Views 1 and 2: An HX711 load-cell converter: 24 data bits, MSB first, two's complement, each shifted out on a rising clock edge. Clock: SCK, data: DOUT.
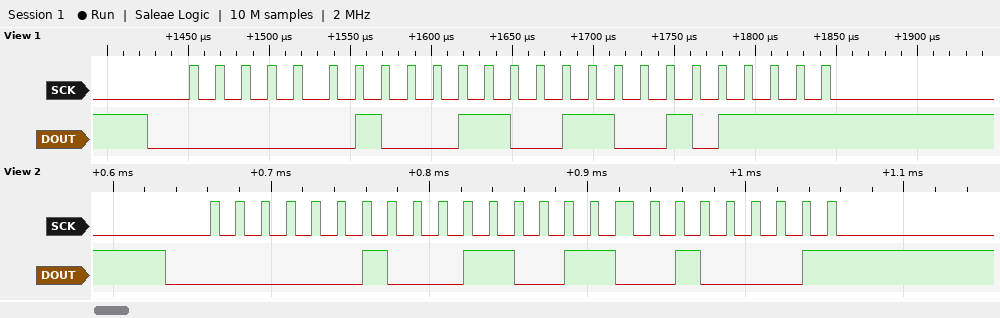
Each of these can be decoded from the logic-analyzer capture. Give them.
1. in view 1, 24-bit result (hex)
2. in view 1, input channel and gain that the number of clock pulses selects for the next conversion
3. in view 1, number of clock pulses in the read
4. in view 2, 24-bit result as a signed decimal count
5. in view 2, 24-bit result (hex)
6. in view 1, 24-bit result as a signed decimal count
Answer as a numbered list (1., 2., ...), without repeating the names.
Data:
1. 0x02332F
2. channel A, gain 128
3. 25
4. 144161
5. 0x023321
6. 144175
